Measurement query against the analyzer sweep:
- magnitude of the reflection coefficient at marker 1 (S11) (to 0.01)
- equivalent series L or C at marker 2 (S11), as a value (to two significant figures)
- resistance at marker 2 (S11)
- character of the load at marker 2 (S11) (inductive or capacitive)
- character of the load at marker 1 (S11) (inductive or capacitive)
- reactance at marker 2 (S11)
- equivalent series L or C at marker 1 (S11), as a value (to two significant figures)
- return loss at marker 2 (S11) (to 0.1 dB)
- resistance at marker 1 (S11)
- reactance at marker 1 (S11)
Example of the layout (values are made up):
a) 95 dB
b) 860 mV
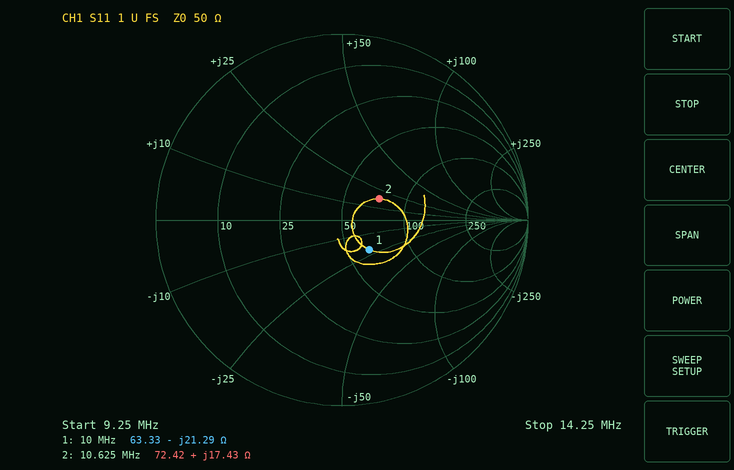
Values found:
a) 0.22
b) 260 nH
c) 72.42 Ω
d) inductive
e) capacitive
f) +17.43 Ω
g) 750 pF
h) 12.8 dB
i) 63.33 Ω
j) -21.29 Ω
